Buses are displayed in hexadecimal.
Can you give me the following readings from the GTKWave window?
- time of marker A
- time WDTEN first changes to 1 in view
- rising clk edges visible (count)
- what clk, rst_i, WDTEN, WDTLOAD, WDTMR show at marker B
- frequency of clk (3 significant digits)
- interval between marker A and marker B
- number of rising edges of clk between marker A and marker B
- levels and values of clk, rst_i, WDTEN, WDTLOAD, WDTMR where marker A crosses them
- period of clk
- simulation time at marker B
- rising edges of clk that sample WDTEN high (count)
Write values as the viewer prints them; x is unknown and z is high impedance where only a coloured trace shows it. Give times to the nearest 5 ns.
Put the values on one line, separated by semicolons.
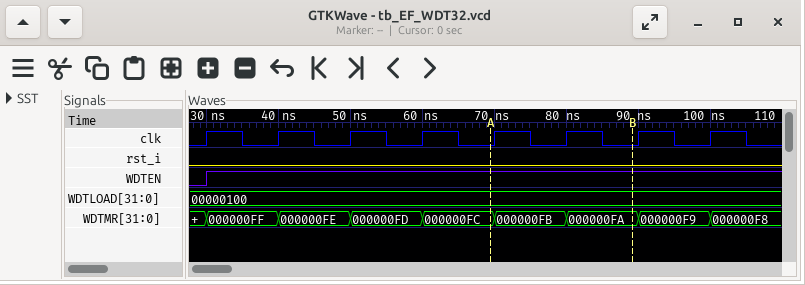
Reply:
70 ns; 30 ns; 8; clk=0, rst_i=0, WDTEN=1, WDTLOAD=00000100, WDTMR=000000FA; 100 MHz; 20 ns; 2; clk=0, rst_i=0, WDTEN=1, WDTLOAD=00000100, WDTMR=000000FC; 10 ns; 90 ns; 7
